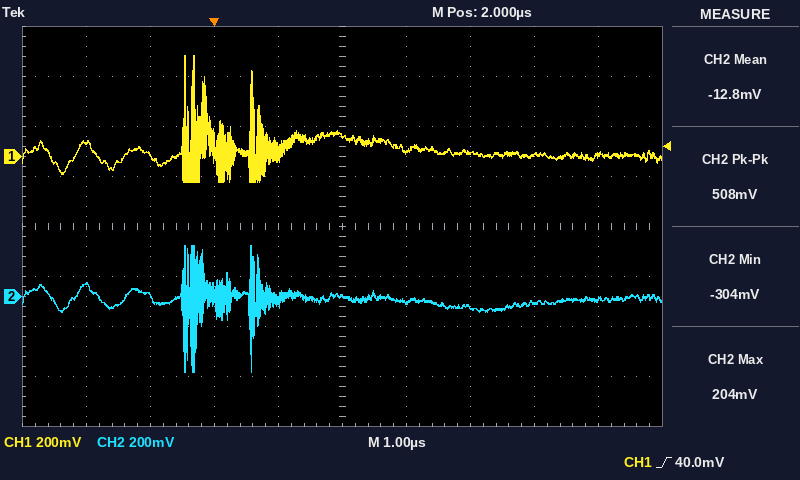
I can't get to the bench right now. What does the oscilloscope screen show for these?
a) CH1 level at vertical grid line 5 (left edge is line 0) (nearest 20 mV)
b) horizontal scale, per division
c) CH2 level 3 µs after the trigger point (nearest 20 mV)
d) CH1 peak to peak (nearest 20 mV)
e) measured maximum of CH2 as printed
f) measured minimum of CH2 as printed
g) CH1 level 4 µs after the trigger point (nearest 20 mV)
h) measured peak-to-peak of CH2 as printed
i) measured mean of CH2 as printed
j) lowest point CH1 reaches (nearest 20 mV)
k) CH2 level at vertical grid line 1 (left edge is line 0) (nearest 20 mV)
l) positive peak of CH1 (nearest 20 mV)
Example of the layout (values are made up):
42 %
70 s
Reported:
80 mV
1 µs
-20 mV
500 mV
204 mV
-304 mV
20 mV
508 mV
-12.8 mV
-100 mV
40 mV
400 mV
